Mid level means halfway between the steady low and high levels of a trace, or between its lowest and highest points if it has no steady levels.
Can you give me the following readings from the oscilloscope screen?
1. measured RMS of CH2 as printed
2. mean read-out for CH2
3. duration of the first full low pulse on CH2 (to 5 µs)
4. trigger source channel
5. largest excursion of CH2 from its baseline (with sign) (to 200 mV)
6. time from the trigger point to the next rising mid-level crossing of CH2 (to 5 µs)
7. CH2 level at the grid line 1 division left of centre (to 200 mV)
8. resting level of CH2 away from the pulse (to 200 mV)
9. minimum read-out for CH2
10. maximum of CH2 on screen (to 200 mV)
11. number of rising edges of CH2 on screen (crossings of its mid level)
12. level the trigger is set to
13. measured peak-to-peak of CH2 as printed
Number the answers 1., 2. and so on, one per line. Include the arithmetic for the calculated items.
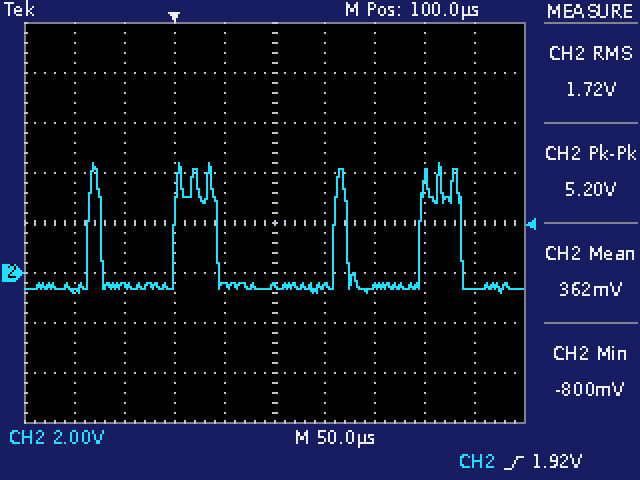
1. 1.72 V
2. 362 mV
3. 75 µs
4. CH2
5. 4.4 V − (-600 mV) = +5.0 V
6. 160 µs
7. -400 mV
8. -600 mV
9. -800 mV
10. 4.4 V
11. 4
12. 1.92 V
13. 5.20 V
